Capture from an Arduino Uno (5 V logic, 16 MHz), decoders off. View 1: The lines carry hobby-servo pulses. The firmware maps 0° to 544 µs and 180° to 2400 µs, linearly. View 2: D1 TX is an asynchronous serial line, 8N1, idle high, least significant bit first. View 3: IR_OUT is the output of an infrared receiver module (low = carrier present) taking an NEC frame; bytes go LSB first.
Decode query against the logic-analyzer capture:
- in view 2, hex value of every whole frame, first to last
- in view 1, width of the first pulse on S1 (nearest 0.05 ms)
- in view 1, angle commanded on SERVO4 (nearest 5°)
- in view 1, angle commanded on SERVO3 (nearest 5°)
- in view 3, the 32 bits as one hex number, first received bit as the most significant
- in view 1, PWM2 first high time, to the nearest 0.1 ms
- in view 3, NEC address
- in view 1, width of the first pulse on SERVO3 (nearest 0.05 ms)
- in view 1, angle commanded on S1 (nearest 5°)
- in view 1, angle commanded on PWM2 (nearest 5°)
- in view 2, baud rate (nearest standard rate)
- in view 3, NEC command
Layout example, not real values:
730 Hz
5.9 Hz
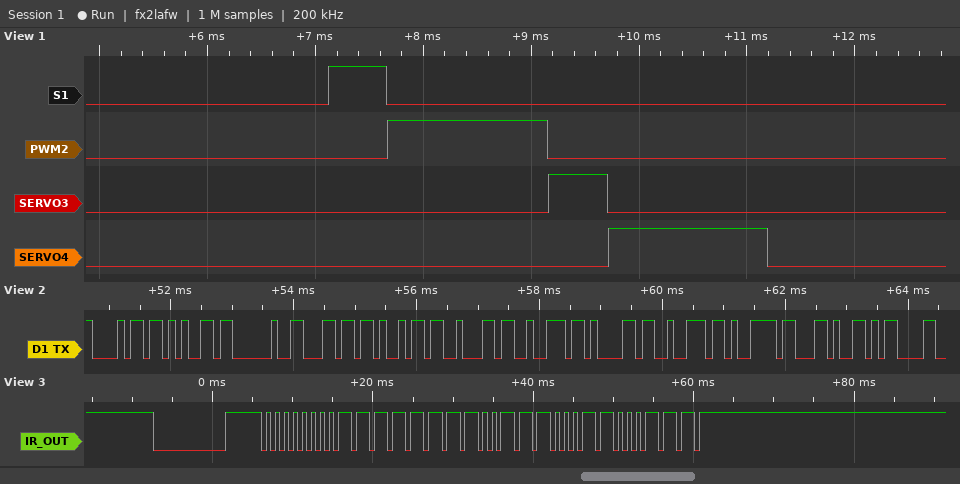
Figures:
68 65 20 6C 69 62 72 61 72 79 2C 0D
0.55 ms
90°
0°
0x00FF38C7
1.5 ms
0x00
0.55 ms
0°
90°
9600 baud
0x1C
